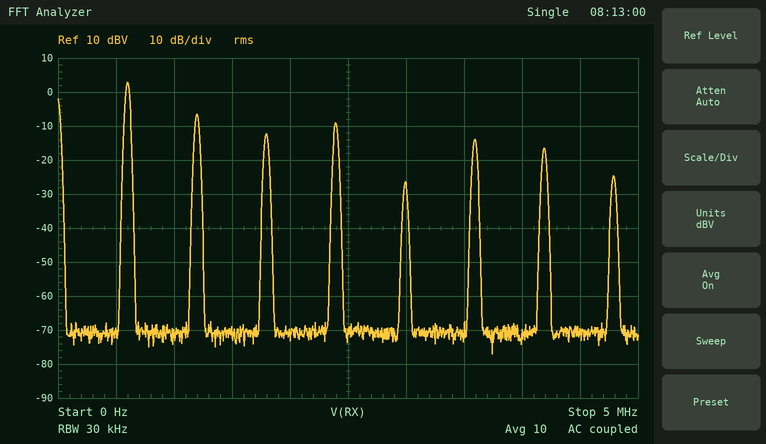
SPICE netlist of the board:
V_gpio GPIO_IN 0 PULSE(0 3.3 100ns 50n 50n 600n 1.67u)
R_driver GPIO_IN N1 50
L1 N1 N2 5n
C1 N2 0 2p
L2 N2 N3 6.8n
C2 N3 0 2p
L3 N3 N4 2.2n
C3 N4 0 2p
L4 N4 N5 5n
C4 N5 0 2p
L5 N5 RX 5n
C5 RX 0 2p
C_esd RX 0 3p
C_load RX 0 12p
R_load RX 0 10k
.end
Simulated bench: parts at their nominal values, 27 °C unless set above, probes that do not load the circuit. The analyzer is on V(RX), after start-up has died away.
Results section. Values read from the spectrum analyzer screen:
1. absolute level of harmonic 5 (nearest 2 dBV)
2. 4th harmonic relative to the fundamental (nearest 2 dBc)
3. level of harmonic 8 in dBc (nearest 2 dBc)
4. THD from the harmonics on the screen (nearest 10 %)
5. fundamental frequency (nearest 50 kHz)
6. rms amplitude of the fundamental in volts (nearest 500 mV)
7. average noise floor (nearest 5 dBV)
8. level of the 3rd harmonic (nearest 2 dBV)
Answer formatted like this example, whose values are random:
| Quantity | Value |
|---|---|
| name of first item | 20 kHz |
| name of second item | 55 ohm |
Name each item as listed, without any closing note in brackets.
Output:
| Quantity | Value |
|---|---|
| absolute level of harmonic 5 | -26 dBV |
| 4th harmonic relative to the fundamental | -12 dBc |
| level of harmonic 8 in dBc | -28 dBc |
| THD from the harmonics on the screen | 50 % |
| fundamental frequency | 600 kHz |
| rms amplitude of the fundamental in volts | 1.5 V |
| average noise floor | -70 dBV |
| level of the 3rd harmonic | -12 dBV |
